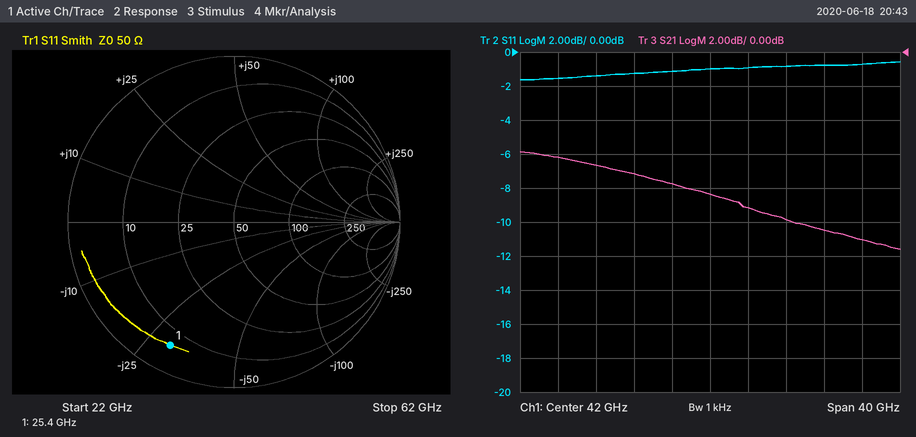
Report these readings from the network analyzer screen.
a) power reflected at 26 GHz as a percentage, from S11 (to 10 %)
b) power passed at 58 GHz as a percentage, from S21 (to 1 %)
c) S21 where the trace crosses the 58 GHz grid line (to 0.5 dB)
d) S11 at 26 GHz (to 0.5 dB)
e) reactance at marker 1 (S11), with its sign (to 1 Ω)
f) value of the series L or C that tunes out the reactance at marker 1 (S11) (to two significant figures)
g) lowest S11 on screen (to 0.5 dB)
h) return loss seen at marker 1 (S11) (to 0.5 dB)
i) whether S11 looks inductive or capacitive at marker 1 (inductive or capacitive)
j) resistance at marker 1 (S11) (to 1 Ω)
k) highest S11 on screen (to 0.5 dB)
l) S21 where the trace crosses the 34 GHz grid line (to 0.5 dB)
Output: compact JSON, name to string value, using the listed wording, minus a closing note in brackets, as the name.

{"power reflected at 26 GHz as a percentage, from S11": "70 %", "power passed at 58 GHz as a percentage, from S21": "8 %", "S21 where the trace crosses the 58 GHz grid line": "-11.0 dB", "S11 at 26 GHz": "-1.5 dB", "reactance at marker 1 (S11), with its sign": "-30 Ω", "value of the series L or C that tunes out the reactance at marker 1 (S11)": "190 pH", "lowest S11 on screen": "-1.5 dB", "return loss seen at marker 1 (S11)": "1.5 dB", "whether S11 looks inductive or capacitive at marker 1": "capacitive", "resistance at marker 1 (S11)": "6 Ω", "highest S11 on screen": "-0.5 dB", "S21 where the trace crosses the 34 GHz grid line": "-7.0 dB"}
